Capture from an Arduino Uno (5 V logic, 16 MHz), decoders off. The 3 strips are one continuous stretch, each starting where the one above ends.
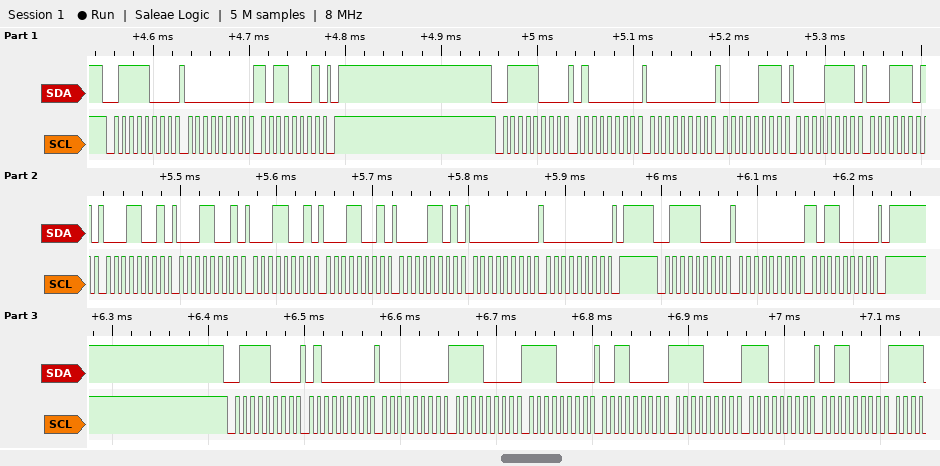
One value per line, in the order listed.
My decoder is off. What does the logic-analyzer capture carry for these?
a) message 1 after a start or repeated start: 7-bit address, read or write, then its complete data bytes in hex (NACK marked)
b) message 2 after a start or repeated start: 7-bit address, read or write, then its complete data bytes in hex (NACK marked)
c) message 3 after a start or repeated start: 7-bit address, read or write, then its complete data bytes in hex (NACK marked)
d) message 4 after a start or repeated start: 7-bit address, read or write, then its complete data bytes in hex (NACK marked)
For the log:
0x3C write: 00 B1
0x3C write: 40 00 07 0F 1D 19 19 19 19 0D 00 00
0x3C write: 00 B0
0x3C write: 40 00 F0 F0 30 F0 E0 30
